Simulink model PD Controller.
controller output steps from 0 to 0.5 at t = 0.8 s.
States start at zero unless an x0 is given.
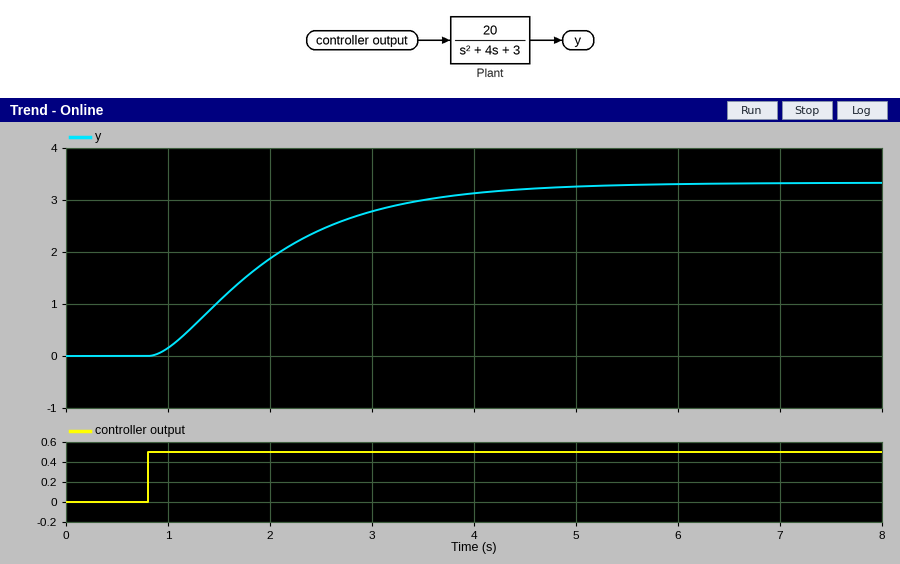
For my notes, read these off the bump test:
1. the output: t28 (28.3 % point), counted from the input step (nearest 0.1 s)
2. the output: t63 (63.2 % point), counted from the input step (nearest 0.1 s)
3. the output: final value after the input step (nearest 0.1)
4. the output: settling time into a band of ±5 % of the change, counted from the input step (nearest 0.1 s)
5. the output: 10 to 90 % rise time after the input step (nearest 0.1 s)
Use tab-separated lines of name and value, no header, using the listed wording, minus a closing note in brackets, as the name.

the output: t28 (28.3 % point), counted from the input step	0.6 s
the output: t63 (63.2 % point), counted from the input step	1.4 s
the output: final value after the input step	3.3
the output: settling time into a band of ±5 % of the change, counted from the input step	3.4 s
the output: 10 to 90 % rise time after the input step	2.4 s
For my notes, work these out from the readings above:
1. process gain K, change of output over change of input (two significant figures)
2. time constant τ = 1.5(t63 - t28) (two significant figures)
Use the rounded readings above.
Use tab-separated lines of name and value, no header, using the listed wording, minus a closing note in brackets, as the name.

process gain K, change of output over change of input	6.6
time constant τ = 1.5(t63 - t28)	1.2 s
